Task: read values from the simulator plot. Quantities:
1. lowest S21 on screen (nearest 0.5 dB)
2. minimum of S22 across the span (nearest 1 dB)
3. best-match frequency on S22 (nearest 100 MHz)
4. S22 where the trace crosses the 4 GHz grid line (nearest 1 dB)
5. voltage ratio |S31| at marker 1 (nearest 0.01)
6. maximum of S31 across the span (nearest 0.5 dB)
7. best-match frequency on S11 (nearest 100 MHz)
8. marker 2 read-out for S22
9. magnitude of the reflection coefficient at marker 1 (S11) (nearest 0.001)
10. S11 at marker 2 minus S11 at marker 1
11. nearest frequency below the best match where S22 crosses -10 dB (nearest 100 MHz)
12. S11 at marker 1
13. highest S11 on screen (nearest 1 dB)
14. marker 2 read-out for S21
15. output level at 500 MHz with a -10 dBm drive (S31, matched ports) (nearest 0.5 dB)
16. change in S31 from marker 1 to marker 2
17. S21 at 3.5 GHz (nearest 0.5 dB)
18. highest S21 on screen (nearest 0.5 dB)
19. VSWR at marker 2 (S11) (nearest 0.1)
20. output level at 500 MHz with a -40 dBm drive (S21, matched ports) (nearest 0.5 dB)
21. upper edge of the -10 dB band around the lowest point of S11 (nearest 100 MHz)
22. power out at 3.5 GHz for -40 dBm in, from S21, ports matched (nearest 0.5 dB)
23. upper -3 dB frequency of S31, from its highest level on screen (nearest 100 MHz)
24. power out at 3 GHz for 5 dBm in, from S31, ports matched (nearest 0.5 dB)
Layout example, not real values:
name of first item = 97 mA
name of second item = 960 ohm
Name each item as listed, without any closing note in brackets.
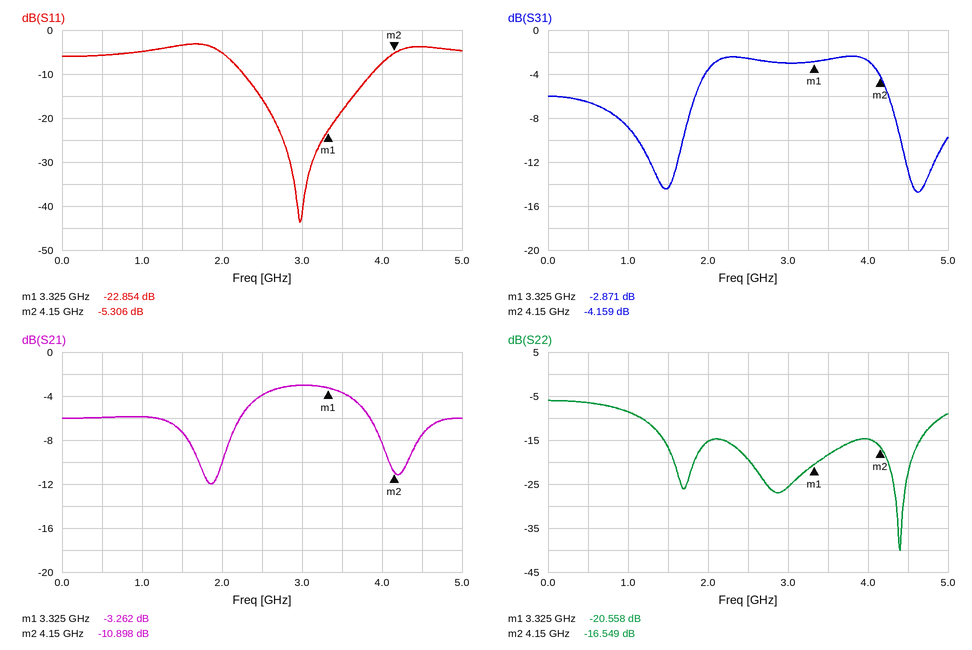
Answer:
lowest S21 on screen = -12.0 dB
minimum of S22 across the span = -40 dB
best-match frequency on S22 = 4.4 GHz
S22 where the trace crosses the 4 GHz grid line = -15 dB
voltage ratio |S31| at marker 1 = 0.72
maximum of S31 across the span = -2.5 dB
best-match frequency on S11 = 3.0 GHz
marker 2 read-out for S22 = -16.549 dB
magnitude of the reflection coefficient at marker 1 (S11) = 0.072
S11 at marker 2 minus S11 at marker 1 = 17.548 dB
nearest frequency below the best match where S22 crosses -10 dB = 1.2 GHz
S11 at marker 1 = -22.854 dB
highest S11 on screen = -3 dB
marker 2 read-out for S21 = -10.898 dB
output level at 500 MHz with a -10 dBm drive (S31, matched ports) = -16.5 dBm
change in S31 from marker 1 to marker 2 = -1.288 dB
S21 at 3.5 GHz = -3.5 dB
highest S21 on screen = -3.0 dB
VSWR at marker 2 (S11) = 3.4
output level at 500 MHz with a -40 dBm drive (S21, matched ports) = -46.0 dBm
upper edge of the -10 dB band around the lowest point of S11 = 3.9 GHz
power out at 3.5 GHz for -40 dBm in, from S21, ports matched = -43.5 dBm
upper -3 dB frequency of S31, from its highest level on screen = 4.2 GHz
power out at 3 GHz for 5 dBm in, from S31, ports matched = 2.0 dBm
